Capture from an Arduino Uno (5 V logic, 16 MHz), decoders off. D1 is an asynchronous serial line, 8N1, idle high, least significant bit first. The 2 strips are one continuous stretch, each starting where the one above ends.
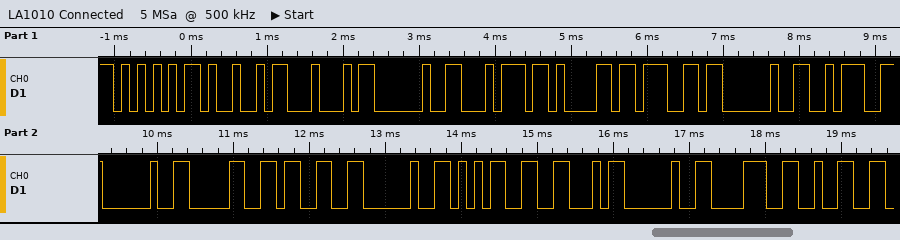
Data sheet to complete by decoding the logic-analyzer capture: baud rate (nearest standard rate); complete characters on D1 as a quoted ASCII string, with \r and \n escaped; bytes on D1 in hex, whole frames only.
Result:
9600 baud
"UID tag : 03 5F 82"
0x55 0x49 0x44 0x20 0x74 0x61 0x67 0x20 0x3A 0x20 0x30 0x33 0x20 0x35 0x46 0x20 0x38 0x32
